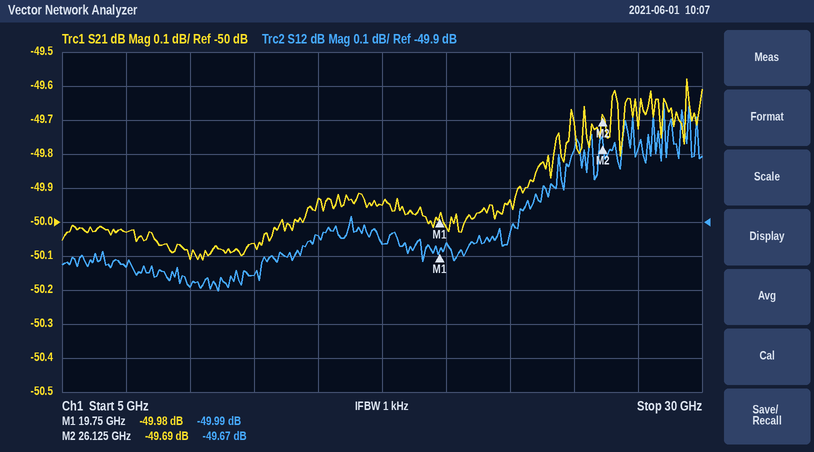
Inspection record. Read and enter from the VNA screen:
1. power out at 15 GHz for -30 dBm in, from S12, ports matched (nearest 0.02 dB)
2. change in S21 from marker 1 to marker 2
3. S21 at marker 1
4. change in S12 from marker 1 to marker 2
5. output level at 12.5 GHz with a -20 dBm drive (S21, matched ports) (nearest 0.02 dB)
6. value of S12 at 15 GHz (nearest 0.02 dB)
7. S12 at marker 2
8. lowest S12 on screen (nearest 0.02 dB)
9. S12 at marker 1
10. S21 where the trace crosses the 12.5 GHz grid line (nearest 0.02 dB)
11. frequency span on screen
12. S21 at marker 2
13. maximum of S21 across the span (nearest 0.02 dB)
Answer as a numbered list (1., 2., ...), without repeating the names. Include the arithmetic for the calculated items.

1. -30 dBm + (-49.94 dB) = -79.94 dBm
2. -49.69 − (-49.98) = 0.29 dB
3. -49.98 dB
4. -49.67 − (-49.99) = 0.32 dB
5. -20 dBm + (-50.06 dB) = -70.06 dBm
6. -49.94 dB
7. -49.67 dB
8. -50.10 dB
9. -49.99 dB
10. -50.06 dB
11. 25 GHz
12. -49.69 dB
13. -49.58 dB
